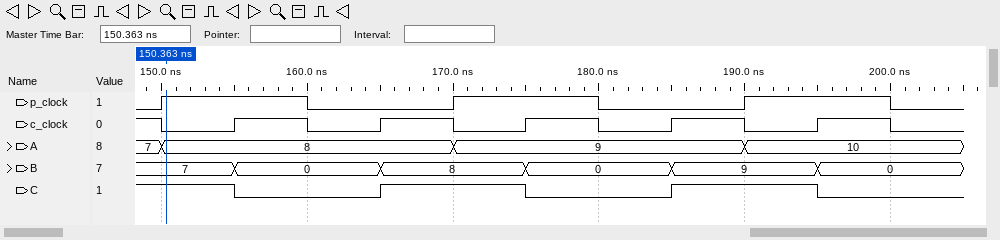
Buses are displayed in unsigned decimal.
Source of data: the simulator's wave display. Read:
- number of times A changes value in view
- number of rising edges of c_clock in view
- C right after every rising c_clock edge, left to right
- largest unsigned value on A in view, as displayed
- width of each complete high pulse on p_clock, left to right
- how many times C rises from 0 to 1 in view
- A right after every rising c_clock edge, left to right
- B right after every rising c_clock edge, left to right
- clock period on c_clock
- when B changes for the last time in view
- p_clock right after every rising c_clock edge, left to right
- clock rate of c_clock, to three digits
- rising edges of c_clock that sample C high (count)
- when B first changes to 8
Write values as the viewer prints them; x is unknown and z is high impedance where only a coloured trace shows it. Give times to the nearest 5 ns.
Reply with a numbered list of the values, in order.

1. 3
2. 5
3. 0 1 0 1 0
4. 10
5. 10 ns, 10 ns, 10 ns
6. 2
7. 8, 8, 9, 9, 10
8. 0, 8, 0, 9, 0
9. 10 ns
10. 195 ns
11. 1 0 1 0 1
12. 100 MHz
13. 3
14. 165 ns
